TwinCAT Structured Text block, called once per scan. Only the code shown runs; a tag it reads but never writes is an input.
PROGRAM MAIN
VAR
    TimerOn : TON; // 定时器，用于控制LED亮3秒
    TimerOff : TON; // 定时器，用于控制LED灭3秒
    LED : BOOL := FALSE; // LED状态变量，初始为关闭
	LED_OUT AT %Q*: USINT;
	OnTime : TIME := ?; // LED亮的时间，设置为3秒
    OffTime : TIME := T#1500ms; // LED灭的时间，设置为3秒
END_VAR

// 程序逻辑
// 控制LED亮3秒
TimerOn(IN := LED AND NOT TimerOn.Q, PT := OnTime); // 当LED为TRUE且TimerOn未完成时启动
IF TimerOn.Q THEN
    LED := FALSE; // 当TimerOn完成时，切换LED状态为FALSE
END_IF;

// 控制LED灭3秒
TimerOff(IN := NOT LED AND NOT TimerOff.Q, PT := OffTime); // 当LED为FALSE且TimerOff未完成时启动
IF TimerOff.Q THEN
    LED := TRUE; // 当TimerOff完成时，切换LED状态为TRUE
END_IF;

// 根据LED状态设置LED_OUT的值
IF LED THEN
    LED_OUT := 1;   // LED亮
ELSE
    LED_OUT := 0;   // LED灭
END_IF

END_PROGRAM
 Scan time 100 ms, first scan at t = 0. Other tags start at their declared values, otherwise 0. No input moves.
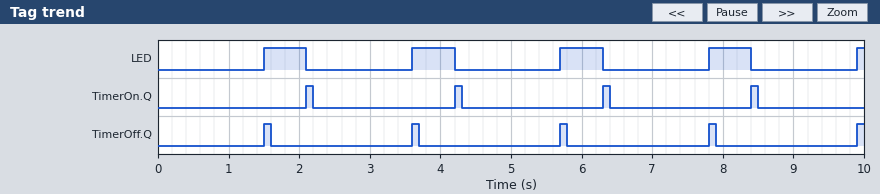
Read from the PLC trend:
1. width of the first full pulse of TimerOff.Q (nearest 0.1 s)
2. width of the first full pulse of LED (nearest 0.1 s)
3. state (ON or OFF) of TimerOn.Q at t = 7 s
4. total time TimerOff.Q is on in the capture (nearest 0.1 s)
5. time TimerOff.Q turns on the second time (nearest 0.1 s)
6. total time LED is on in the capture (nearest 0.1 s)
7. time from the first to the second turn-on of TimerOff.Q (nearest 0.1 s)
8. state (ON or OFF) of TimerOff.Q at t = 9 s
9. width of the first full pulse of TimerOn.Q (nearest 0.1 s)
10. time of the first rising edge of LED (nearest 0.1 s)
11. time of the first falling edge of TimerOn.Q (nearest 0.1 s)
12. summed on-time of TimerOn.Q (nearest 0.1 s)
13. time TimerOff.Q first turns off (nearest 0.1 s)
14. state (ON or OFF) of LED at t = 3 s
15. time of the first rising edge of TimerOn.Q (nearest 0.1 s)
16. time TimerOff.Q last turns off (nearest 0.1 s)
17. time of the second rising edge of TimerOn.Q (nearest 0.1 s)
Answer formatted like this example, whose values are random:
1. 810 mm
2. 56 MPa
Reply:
1. 0.1 s
2. 0.6 s
3. OFF
4. 0.5 s
5. 3.6 s
6. 2.5 s
7. 2.1 s
8. OFF
9. 0.1 s
10. 1.5 s
11. 2.2 s
12. 0.4 s
13. 1.6 s
14. OFF
15. 2.1 s
16. 7.9 s
17. 4.2 s
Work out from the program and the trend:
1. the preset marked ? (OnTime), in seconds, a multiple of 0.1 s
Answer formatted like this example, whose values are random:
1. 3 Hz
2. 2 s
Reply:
1. 0.5 s
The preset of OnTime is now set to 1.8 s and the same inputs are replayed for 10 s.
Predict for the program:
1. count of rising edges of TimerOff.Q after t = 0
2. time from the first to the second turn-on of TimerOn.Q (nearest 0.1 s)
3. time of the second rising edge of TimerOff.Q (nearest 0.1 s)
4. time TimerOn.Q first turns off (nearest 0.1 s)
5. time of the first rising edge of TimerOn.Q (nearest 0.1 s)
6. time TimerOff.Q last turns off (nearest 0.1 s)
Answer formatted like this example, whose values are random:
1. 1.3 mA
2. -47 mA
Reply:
1. 3
2. 3.4 s
3. 4.9 s
4. 3.5 s
5. 3.4 s
6. 8.4 s
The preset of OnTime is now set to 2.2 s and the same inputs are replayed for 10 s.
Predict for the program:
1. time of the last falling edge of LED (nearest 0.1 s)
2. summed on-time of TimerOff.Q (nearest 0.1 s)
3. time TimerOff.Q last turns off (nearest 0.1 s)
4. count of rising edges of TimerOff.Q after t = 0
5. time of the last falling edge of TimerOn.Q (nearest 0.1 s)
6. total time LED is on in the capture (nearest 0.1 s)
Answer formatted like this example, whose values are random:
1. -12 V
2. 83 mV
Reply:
1. 7.6 s
2. 0.3 s
3. 9.2 s
4. 3
5. 7.7 s
6. 5.5 s
